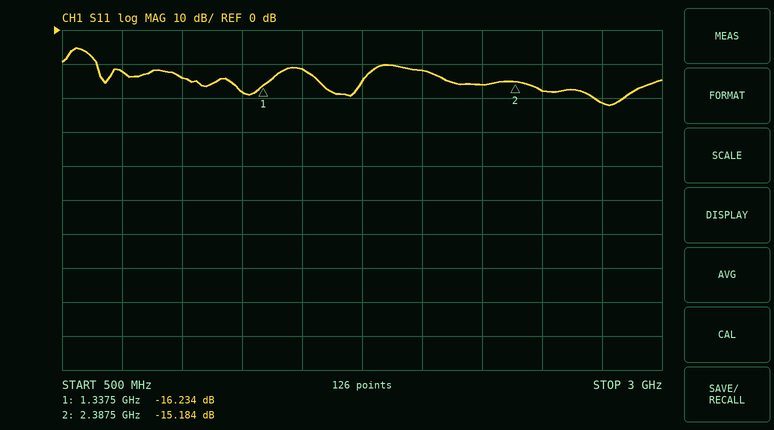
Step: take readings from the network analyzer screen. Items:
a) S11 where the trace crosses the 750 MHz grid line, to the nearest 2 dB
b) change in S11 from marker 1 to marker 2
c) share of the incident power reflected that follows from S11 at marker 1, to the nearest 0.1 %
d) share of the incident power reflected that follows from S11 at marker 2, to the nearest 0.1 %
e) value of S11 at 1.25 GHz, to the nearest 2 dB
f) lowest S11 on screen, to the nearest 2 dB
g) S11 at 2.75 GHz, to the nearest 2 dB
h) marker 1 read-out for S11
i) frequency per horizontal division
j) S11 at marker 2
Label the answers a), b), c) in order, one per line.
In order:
a) -12 dB
b) 1.050 dB
c) 2.4 %
d) 3.0 %
e) -18 dB
f) -22 dB
g) -22 dB
h) -16.234 dB
i) 250 MHz
j) -15.184 dB
